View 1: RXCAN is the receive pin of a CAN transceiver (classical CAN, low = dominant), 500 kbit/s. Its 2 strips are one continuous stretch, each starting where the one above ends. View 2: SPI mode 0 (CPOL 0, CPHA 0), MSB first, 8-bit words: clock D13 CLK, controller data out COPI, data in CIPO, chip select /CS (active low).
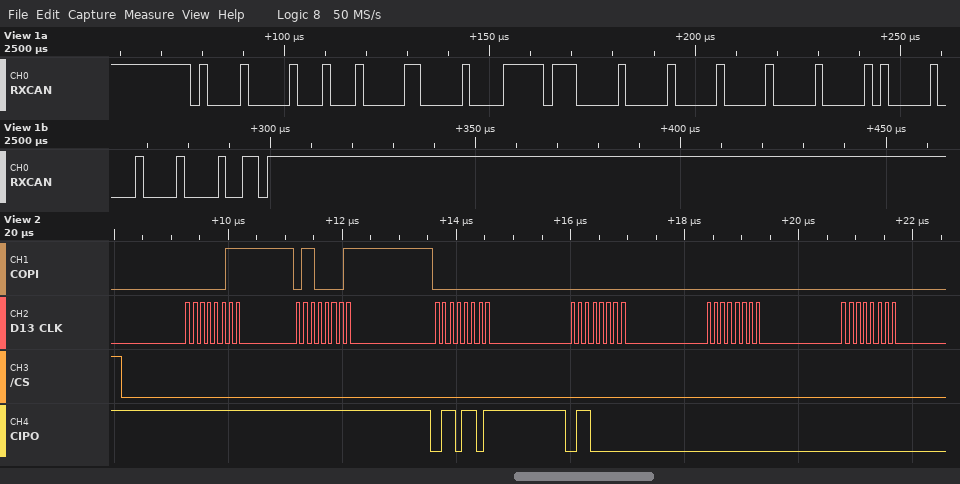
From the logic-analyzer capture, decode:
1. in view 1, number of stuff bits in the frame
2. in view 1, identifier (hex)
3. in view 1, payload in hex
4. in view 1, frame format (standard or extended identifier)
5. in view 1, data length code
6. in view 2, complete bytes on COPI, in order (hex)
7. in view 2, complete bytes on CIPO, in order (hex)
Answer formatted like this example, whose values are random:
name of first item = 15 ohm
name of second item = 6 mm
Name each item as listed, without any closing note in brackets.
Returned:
in view 1, number of stuff bits in the frame = 11
in view 1, identifier = 0x420
in view 1, payload in hex = 82 00 FF 00 00 00 01 00
in view 1, frame format = standard
in view 1, data length code = 8
in view 2, complete bytes on COPI, in order = 03 61 00 00 00 00
in view 2, complete bytes on CIPO, in order = FF FF 6D 60 00 00
